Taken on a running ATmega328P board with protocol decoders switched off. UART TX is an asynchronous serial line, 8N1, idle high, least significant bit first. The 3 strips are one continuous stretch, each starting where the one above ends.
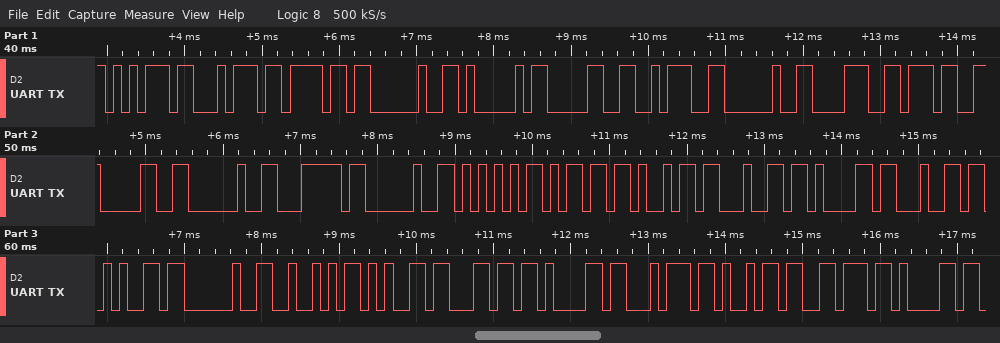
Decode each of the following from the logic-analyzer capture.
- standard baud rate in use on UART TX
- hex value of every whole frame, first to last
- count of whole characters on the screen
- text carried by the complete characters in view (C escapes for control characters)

9600 baud
0x75 0x74 0x6F 0x20 0x41 0x30 0x3A 0x20 0x38 0x37 0x30 0x20 0x7C 0x20 0x55 0x6D 0x69 0x64 0x61 0x64 0x65 0x20 0x52 0x65 0x6C 0x61 0x74 0x69 0x76 0x61
30
"uto A0: 870 | Umidade Relativa"
